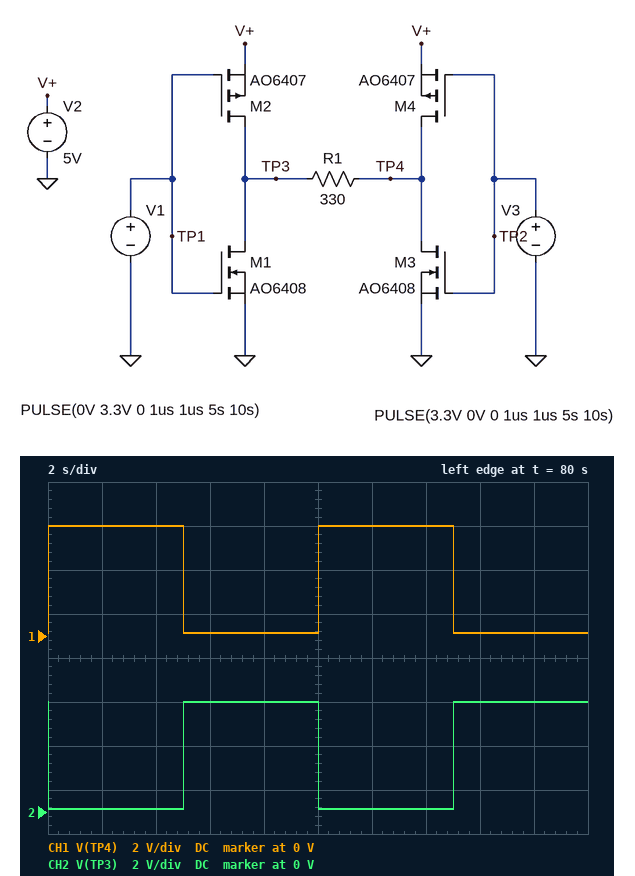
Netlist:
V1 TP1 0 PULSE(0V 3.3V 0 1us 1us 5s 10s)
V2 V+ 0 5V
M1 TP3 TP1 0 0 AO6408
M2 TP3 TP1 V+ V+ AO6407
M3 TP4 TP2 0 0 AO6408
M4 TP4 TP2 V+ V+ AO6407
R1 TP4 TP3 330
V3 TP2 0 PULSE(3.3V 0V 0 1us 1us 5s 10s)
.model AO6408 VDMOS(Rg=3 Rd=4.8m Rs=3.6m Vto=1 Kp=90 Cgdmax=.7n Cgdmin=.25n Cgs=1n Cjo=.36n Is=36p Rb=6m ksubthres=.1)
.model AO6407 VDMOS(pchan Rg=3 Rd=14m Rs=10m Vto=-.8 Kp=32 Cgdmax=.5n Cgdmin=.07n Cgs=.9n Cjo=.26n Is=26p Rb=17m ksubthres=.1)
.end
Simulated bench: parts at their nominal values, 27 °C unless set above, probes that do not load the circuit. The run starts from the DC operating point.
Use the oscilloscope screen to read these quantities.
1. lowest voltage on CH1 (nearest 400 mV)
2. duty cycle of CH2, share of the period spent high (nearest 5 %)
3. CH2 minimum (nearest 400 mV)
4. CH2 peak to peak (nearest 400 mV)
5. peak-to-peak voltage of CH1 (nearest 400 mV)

0 V
50 %
0 V
4.8 V
4.8 V
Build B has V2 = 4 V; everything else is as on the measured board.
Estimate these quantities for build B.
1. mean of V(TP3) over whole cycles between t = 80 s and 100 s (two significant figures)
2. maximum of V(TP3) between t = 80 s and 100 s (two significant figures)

2.0 V
4.0 V
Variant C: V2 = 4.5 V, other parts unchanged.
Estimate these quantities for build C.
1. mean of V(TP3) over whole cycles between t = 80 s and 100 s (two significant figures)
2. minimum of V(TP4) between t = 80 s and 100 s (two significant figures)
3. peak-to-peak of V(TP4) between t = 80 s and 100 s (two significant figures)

2.3 V
31 mV
4.5 V
